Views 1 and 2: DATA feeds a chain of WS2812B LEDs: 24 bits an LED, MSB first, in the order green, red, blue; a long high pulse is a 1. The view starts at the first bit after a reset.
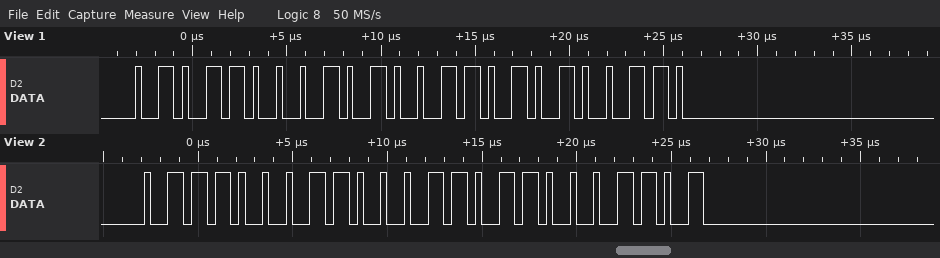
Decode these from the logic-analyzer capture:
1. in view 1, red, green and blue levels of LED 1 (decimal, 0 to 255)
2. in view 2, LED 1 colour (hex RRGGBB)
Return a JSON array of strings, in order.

["166, 88, 166", "#8D718D"]
